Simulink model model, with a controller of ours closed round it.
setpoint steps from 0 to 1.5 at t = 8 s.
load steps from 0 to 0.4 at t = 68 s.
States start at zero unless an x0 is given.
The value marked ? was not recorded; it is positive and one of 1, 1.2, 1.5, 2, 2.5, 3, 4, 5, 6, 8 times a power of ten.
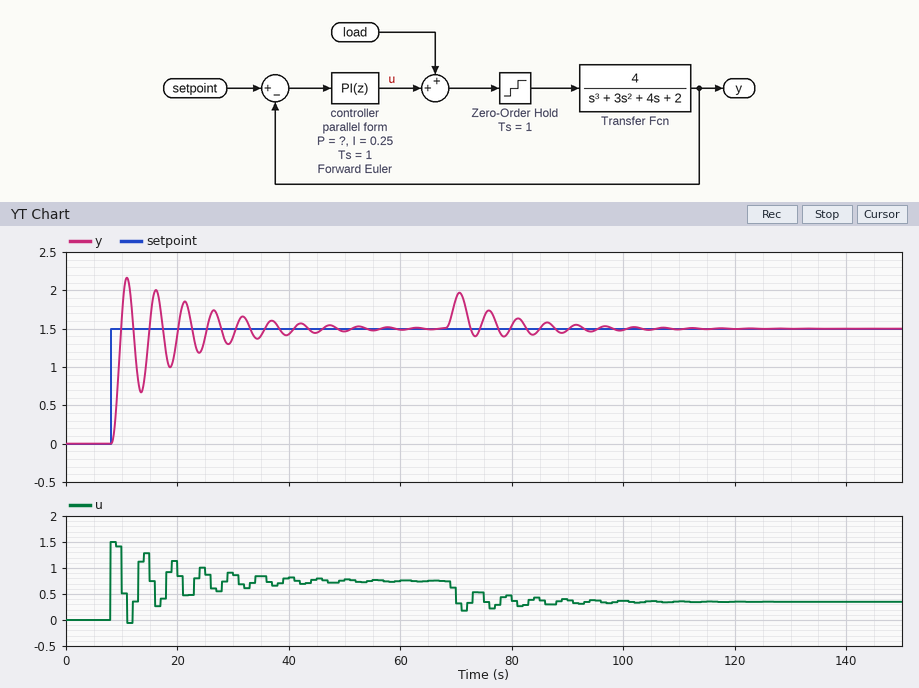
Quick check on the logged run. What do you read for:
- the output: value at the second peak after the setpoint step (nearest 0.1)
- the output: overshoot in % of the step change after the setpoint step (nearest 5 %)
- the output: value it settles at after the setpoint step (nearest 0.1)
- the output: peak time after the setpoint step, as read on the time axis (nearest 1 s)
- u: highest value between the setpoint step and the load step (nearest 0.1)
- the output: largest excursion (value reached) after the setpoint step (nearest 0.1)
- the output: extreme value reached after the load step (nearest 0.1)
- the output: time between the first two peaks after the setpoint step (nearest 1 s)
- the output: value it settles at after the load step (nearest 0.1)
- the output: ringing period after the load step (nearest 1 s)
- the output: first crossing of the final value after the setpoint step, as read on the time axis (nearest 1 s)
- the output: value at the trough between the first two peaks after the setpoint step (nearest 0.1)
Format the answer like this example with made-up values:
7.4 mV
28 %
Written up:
2.0
45 %
1.5
11 s
1.5
2.2
2.0
5 s
1.5
5 s
10 s
0.7
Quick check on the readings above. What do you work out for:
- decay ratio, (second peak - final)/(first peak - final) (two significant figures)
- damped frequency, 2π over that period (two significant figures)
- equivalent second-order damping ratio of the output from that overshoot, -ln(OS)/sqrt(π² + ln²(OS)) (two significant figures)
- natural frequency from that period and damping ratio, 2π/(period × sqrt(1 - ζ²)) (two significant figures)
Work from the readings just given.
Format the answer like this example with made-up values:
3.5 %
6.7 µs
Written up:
0.71
1.3 rad/s
0.25
1.3 rad/s
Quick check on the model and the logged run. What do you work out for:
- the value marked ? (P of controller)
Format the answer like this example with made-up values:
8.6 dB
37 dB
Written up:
1
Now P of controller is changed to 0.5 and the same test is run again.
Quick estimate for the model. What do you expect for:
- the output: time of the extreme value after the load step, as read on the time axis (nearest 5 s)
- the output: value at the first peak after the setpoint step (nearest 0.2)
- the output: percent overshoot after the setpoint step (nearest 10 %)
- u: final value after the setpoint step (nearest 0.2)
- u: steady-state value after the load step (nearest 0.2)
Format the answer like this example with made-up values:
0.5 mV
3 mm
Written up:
70 s
1.8
20 %
0.8
0.4
